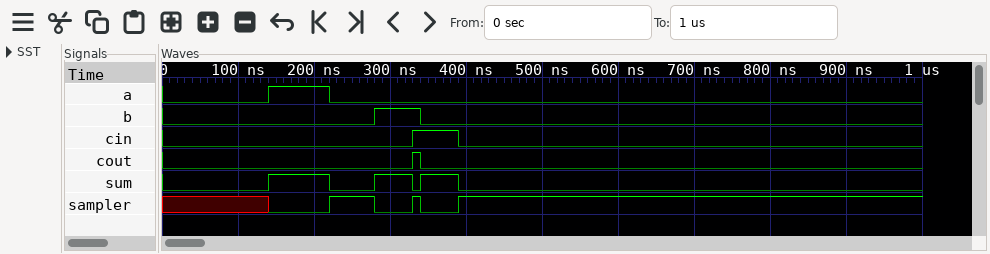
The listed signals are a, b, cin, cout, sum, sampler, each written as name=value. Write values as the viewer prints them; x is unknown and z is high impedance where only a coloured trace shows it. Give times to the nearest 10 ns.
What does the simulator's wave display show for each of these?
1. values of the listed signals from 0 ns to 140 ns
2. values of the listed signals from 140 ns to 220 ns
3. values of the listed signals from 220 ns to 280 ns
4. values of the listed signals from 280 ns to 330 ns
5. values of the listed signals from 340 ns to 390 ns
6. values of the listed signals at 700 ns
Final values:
a=0, b=0, cin=0, cout=0, sum=0, sampler=x
a=1, b=0, cin=0, cout=0, sum=1, sampler=0
a=0, b=0, cin=0, cout=0, sum=0, sampler=1
a=0, b=1, cin=0, cout=0, sum=1, sampler=0
a=0, b=0, cin=1, cout=0, sum=1, sampler=0
a=0, b=0, cin=0, cout=0, sum=0, sampler=1
